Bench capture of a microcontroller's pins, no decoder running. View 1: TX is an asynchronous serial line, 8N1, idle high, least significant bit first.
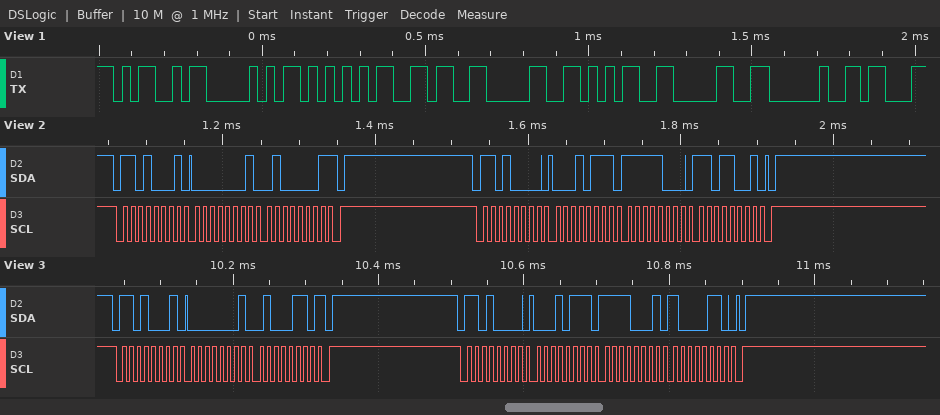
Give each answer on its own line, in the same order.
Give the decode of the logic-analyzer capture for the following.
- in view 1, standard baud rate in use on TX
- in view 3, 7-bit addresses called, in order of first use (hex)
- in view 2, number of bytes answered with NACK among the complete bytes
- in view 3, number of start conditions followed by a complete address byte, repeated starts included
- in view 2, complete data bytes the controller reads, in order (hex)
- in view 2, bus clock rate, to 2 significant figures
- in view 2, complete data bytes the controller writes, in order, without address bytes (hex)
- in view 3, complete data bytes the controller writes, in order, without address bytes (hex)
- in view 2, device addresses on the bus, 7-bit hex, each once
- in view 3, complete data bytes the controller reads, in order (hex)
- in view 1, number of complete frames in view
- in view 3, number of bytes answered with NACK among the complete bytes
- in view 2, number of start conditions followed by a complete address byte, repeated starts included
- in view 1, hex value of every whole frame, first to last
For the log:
38400 baud
0x68
1
2
01 41
100 kHz
17 F8 D9
17 F1 86
0x68
01 46
8
1
2
0x4D 0x50 0x55 0x36 0x30 0x35 0x30 0x20
